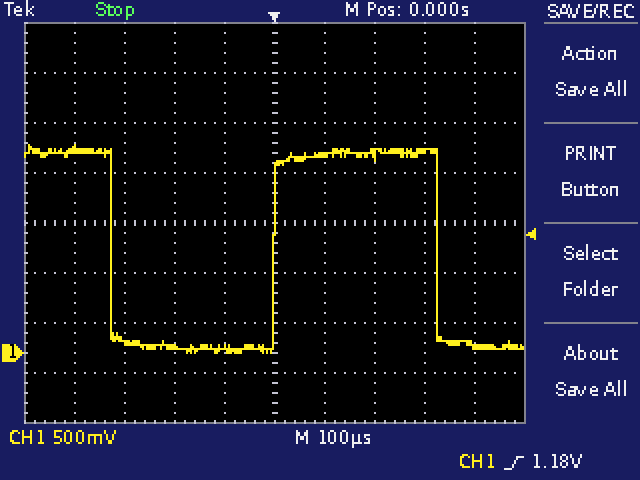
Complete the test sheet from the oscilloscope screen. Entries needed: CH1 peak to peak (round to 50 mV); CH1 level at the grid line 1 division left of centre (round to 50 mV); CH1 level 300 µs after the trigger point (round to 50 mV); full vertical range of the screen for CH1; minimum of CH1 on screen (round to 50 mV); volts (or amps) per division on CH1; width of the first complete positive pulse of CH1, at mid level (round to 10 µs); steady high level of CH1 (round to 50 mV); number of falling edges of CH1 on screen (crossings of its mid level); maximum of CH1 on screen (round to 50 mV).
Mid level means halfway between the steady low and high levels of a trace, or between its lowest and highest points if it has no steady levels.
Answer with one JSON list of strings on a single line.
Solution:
["2.10 V", "50 mV", "2.00 V", "4 V", "0 mV", "500 mV", "330 µs", "2.00 V", "2", "2.10 V"]
